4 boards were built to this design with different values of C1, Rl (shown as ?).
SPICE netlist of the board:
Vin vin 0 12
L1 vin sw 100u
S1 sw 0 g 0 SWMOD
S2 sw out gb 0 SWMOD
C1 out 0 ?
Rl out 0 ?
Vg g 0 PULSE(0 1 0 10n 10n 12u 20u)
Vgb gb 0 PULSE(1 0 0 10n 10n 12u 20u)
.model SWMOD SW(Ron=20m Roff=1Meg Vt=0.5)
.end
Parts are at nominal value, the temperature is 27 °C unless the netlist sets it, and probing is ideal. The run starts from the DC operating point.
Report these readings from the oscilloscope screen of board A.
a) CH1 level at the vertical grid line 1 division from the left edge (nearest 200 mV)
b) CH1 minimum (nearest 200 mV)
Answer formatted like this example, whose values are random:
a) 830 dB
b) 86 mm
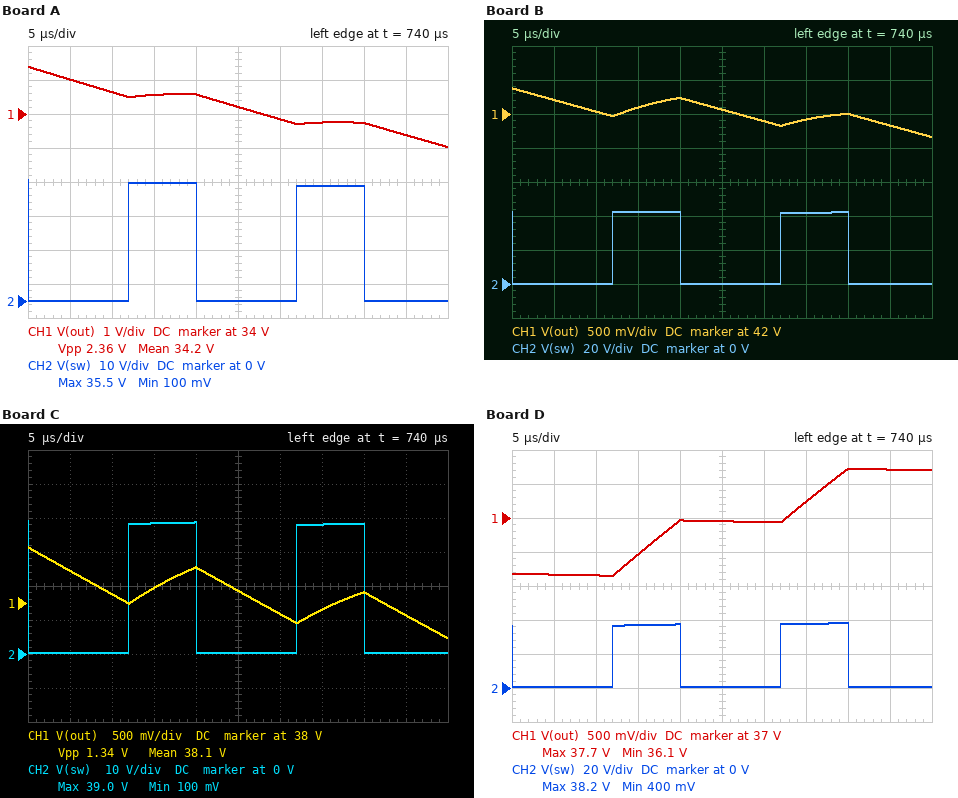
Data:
a) 35.0 V
b) 33.0 V
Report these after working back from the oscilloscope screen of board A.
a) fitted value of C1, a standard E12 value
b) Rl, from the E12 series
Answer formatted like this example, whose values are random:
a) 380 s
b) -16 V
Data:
a) 47 µF
b) 10 Ω
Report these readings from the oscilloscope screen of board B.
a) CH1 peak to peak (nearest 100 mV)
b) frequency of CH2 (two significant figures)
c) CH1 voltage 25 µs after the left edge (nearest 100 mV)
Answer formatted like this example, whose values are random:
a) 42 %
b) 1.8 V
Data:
a) 700 mV
b) 50 kHz
c) 42.1 V
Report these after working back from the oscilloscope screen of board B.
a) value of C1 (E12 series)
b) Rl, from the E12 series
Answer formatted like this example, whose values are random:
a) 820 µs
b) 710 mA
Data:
a) 82 µF
b) 15 Ω
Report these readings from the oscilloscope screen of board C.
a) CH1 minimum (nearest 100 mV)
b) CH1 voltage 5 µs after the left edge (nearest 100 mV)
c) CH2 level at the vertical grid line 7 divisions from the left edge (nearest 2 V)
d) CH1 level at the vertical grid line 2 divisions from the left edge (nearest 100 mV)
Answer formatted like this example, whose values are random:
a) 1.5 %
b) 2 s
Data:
a) 37.5 V
b) 38.5 V
c) 38 V
d) 38.1 V
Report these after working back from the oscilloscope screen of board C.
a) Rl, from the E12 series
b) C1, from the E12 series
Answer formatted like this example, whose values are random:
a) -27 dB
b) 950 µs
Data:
a) 8.2 Ω
b) 68 µF
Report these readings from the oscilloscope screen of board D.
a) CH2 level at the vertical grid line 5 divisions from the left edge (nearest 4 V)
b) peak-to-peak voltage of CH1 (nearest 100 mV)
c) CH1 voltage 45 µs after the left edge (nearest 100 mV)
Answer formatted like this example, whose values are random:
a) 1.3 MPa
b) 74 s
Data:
a) 0 V
b) 1.6 V
c) 37.7 V
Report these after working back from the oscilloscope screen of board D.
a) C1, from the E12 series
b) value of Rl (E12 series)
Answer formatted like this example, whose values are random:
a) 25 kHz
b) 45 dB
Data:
a) 220 µF
b) 68 Ω
